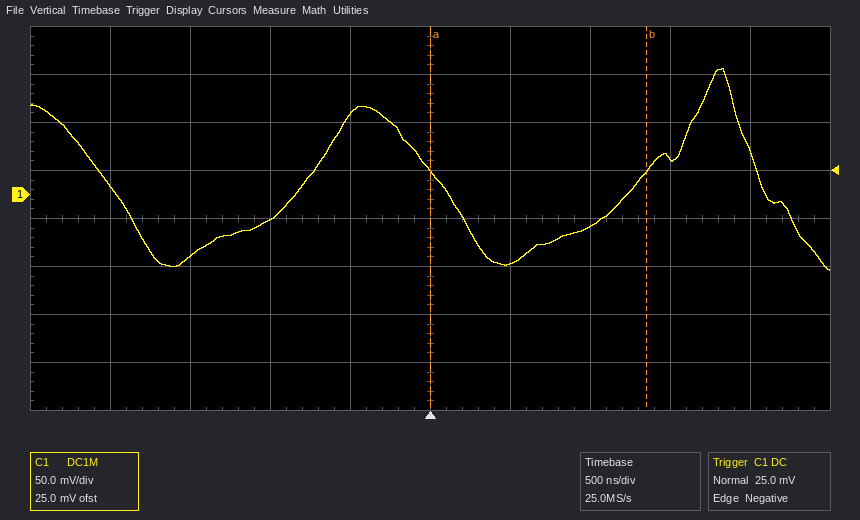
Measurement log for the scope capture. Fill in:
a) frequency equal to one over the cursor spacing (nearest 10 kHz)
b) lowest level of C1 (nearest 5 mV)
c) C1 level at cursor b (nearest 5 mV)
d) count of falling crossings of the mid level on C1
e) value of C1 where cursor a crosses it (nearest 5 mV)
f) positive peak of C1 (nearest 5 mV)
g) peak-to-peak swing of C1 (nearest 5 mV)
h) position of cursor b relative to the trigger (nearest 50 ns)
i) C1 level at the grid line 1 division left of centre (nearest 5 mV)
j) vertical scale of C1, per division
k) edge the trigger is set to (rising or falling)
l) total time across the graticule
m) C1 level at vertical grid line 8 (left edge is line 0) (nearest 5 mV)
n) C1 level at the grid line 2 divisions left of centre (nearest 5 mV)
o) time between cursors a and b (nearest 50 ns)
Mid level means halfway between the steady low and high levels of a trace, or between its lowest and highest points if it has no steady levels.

740 kHz
-80 mV
25 mV
3
25 mV
130 mV
210 mV
+1.35 µs
85 mV
50 mV
falling
5 µs
40 mV
-25 mV
1.35 µs
